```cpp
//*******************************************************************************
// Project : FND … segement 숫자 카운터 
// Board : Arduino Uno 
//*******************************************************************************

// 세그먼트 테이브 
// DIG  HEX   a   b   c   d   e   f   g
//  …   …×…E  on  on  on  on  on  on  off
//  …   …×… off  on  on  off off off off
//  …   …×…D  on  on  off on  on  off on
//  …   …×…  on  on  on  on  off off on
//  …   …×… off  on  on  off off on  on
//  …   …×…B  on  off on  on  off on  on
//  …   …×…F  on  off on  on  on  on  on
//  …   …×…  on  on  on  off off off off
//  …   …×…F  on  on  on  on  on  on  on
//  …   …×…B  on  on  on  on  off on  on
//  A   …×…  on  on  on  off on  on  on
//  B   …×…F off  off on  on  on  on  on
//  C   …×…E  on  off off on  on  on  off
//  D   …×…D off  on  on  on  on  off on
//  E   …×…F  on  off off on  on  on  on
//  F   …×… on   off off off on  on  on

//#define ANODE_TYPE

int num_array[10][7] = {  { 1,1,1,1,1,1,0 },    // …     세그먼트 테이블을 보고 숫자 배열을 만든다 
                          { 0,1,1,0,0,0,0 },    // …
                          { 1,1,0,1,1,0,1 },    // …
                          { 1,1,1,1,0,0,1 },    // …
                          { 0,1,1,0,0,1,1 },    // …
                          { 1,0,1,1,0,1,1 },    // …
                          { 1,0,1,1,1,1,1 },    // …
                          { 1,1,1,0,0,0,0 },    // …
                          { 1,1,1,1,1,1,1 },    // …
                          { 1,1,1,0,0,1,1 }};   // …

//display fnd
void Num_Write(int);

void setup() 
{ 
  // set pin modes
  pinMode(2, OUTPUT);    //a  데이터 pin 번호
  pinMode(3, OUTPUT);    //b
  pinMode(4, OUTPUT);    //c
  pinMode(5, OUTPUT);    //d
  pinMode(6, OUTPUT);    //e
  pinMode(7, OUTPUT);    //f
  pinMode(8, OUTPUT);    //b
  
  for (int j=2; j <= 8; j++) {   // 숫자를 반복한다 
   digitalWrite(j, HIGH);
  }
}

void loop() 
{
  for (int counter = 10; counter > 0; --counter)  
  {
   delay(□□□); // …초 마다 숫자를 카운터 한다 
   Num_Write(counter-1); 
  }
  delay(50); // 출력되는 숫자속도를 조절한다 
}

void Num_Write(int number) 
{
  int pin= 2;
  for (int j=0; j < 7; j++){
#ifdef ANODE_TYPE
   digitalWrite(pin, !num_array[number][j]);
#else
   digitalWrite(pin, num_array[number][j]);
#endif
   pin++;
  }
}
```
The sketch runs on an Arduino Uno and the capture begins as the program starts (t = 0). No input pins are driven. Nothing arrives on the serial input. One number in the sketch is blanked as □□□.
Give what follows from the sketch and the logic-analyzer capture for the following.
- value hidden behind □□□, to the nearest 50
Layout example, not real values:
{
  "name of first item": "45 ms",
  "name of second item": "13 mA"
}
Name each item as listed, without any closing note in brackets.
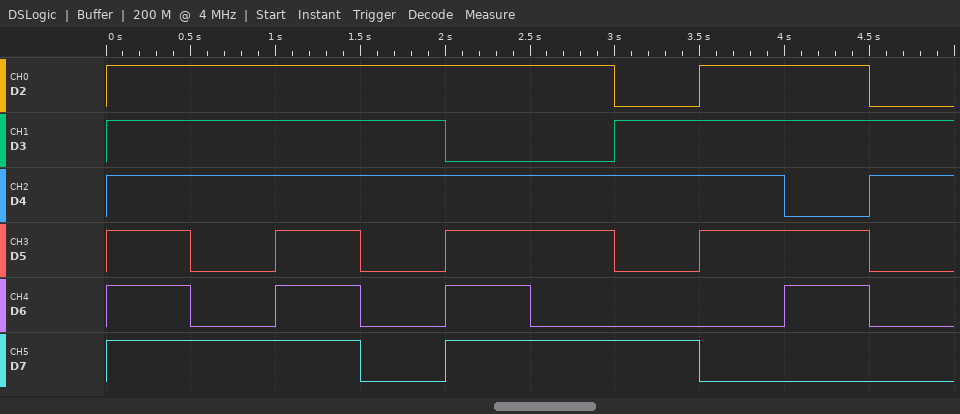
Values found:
{
  "value hidden behind □□□, to the nearest 50": "500"
}
